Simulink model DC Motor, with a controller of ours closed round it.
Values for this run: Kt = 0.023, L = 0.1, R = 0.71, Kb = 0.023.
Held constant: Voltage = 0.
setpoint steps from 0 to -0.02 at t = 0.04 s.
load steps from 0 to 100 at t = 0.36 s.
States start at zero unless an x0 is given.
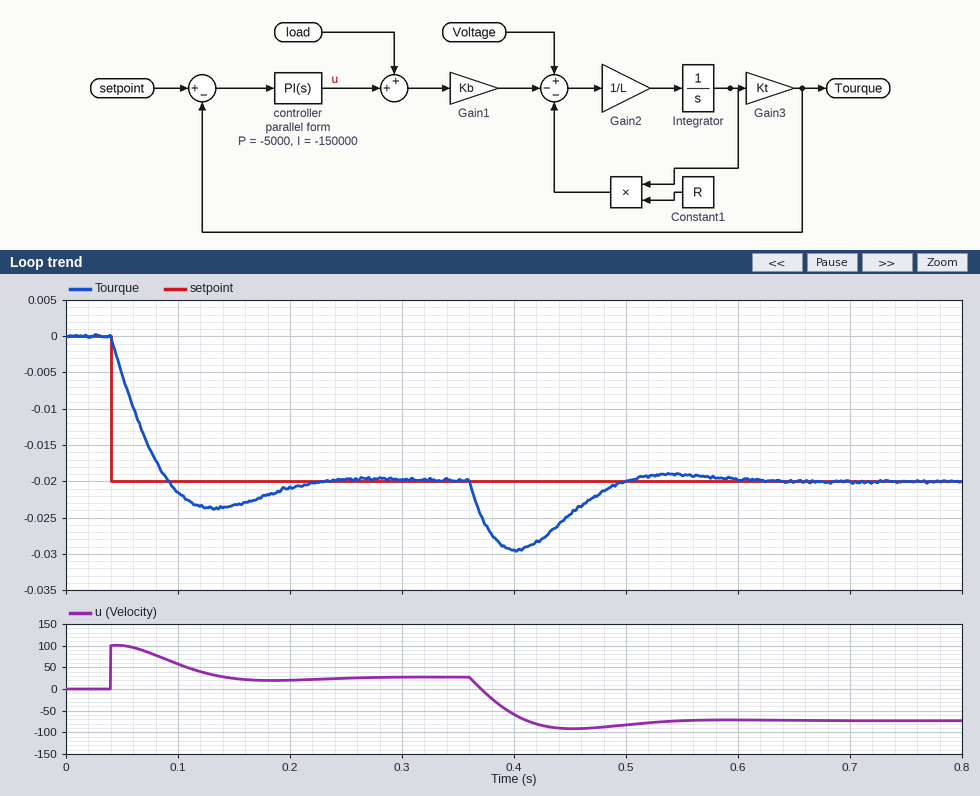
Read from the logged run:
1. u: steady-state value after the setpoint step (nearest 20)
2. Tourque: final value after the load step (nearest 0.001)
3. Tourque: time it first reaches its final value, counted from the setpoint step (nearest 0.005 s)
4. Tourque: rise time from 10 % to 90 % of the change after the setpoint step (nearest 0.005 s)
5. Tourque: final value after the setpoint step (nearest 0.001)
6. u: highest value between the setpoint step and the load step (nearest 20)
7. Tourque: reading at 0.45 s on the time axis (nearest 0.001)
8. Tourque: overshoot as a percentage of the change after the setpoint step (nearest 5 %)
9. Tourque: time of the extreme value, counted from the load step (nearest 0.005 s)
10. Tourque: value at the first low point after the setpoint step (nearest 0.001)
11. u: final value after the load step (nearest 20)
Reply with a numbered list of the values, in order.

1. 20
2. -0.020
3. 0.050 s
4. 0.040 s
5. -0.020
6. 100
7. -0.025
8. 20 %
9. 0.040 s
10. -0.024
11. -80
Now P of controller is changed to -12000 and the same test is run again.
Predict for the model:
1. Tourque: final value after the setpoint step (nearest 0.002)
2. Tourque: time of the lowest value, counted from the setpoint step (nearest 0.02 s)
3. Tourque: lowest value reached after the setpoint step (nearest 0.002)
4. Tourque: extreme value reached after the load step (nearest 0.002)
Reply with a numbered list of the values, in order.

1. -0.020
2. 0.08 s
3. -0.020
4. -0.026
